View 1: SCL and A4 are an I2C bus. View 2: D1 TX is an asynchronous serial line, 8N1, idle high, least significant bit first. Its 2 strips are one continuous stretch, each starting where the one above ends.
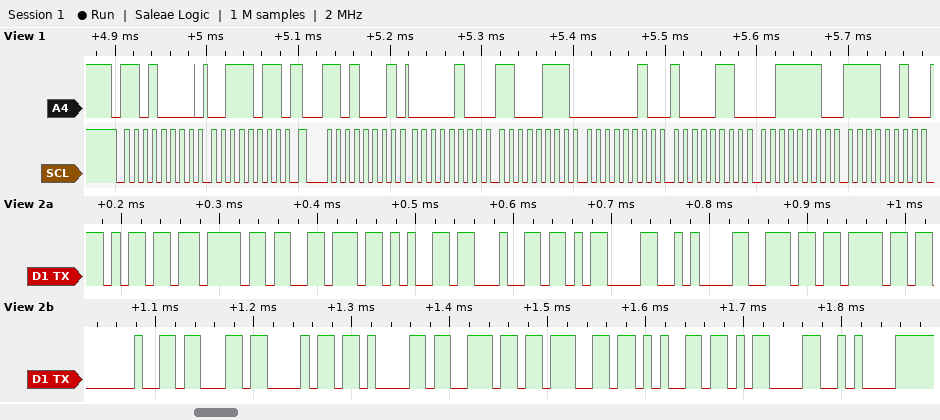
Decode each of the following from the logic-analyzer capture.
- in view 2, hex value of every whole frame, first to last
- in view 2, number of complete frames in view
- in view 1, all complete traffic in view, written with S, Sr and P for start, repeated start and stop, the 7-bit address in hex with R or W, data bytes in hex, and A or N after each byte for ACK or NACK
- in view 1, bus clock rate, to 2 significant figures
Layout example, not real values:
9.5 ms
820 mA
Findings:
6D 6F 76 65 64 0D 0A 6E 6F 20 63 68 61 6E 67 65 0D 0A
18
S 68W A 3B A Sr 68R A 04 A C7 A 02 A 86 A 3E A F2 A
100 kHz
